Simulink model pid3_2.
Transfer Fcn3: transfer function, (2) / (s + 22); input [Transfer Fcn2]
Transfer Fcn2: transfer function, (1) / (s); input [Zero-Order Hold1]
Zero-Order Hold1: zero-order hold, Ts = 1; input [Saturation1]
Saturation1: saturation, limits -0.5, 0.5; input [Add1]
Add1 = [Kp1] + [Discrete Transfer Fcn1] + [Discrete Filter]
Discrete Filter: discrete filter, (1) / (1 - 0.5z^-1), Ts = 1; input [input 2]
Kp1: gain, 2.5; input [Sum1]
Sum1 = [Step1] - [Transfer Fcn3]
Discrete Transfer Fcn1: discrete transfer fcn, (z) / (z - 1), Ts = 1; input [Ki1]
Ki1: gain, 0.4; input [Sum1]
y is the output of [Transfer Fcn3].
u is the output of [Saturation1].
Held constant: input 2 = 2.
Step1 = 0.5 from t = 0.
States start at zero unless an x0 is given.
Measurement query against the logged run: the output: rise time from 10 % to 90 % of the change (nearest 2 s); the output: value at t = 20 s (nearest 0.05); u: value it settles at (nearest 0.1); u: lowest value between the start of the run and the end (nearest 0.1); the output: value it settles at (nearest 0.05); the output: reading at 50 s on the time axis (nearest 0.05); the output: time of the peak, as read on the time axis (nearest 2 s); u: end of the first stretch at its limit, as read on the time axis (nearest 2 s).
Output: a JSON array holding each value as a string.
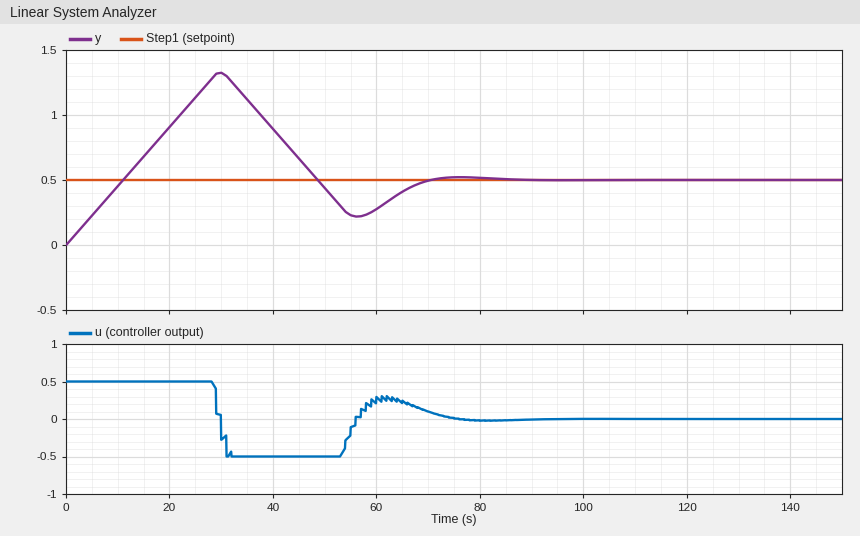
["8 s", "0.90", "0.0", "-0.5", "0.50", "0.45", "30 s", "28 s"]
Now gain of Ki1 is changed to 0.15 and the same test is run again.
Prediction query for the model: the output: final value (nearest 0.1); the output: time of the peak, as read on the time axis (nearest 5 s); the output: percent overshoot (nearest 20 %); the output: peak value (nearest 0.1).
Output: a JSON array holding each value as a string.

["0.5", "35 s", "200 %", "1.5"]
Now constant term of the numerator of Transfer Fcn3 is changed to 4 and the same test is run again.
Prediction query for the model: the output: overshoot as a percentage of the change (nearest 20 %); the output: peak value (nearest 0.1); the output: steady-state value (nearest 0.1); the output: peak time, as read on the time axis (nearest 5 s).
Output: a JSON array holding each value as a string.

["200 %", "1.5", "0.5", "15 s"]
